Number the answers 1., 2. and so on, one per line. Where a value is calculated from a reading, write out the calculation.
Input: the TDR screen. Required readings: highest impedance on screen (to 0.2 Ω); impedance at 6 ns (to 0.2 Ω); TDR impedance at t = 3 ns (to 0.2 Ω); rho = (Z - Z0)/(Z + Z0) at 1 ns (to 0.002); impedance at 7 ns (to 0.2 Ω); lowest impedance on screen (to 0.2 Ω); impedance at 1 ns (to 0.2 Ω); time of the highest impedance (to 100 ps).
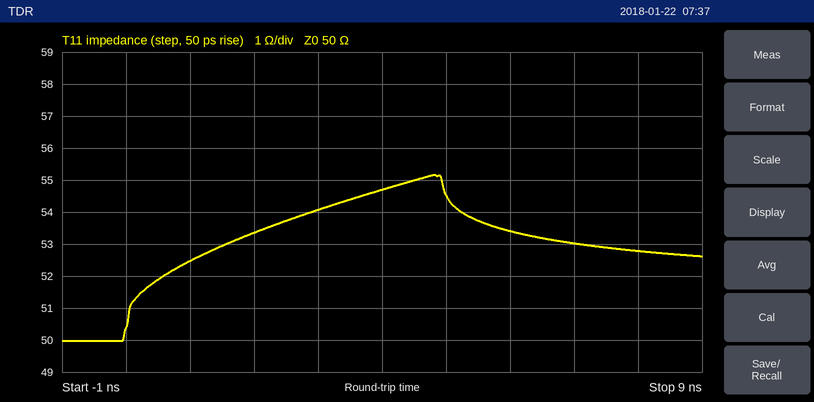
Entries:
1. 55.2 Ω
2. 53.4 Ω
3. 54.0 Ω
4. (52.4 − 50)/(52.4 + 50) ≈ +0.0234, so +0.024 to the nearest 0.002
5. 53.0 Ω
6. 50.0 Ω
7. 52.4 Ω
8. 4.8 ns
